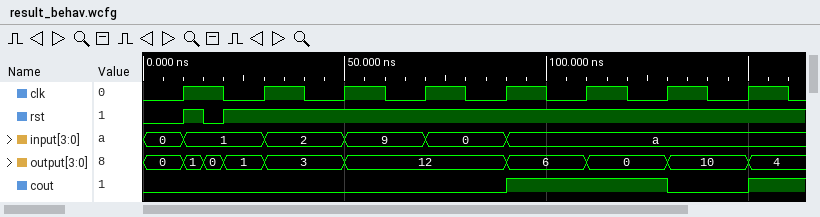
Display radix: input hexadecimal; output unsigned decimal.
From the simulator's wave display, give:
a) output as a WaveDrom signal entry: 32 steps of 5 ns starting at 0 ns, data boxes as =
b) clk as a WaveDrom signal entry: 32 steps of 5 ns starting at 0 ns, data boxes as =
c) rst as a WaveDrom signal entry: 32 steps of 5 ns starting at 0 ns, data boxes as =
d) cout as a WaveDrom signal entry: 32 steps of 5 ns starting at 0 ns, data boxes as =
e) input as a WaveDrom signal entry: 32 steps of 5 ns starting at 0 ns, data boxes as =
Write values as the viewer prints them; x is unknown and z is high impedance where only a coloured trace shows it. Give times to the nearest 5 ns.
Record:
{name: 'output', wave: '=.===.=...=.......=...=...=...=.', data: '0 1 0 1 3 12 6 0 10 4'}
{name: 'clk', wave: '0.1.0.1.0.1.0.1.0.1.0.1.0.1.0.1.'}
{name: 'rst', wave: '0.101...........................'}
{name: 'cout', wave: '0.................1.......0...1.'}
{name: 'input', wave: '=.=...=...=...=...=.............', data: '0 1 2 9 0 a'}
